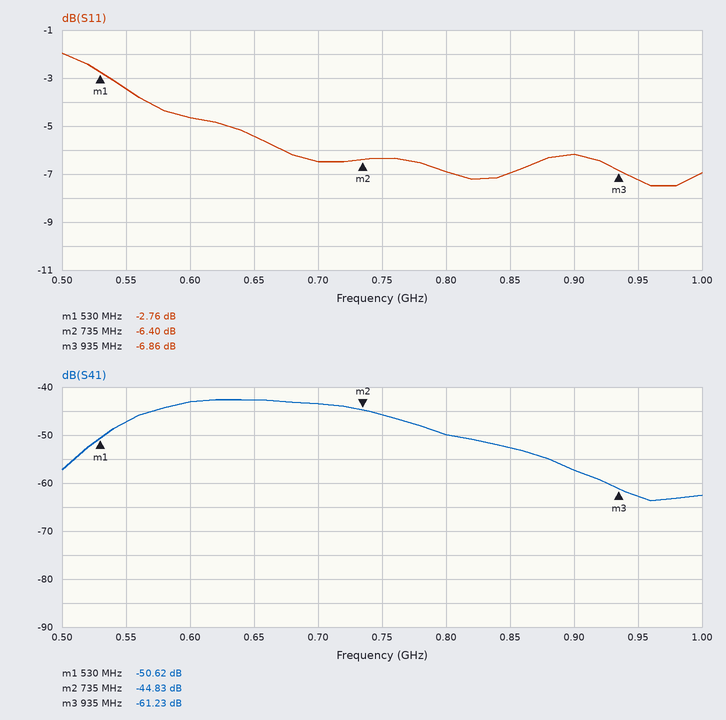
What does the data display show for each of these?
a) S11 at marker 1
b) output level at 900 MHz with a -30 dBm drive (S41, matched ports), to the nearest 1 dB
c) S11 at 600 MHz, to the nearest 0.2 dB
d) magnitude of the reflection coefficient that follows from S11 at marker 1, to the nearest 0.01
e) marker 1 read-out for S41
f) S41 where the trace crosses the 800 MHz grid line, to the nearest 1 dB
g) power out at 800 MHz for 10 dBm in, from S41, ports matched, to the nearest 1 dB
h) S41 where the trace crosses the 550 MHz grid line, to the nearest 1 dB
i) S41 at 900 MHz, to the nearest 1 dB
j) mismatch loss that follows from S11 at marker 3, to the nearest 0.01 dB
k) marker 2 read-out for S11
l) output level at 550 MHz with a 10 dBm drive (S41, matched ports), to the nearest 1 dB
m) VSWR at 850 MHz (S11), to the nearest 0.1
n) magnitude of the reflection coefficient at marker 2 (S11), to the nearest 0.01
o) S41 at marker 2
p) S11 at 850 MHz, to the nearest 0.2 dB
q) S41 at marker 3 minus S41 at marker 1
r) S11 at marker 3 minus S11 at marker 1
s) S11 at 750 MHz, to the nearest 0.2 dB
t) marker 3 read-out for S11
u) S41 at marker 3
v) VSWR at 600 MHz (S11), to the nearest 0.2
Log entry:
-2.76 dB
-87 dBm
-4.6 dB
0.73
-50.62 dB
-50 dB
-40 dBm
-47 dB
-57 dB
1.00 dB
-6.40 dB
-37 dBm
2.6
0.48
-44.83 dB
-7.0 dB
-10.61 dB
-4.10 dB
-6.4 dB
-6.86 dB
-61.23 dB
3.8
